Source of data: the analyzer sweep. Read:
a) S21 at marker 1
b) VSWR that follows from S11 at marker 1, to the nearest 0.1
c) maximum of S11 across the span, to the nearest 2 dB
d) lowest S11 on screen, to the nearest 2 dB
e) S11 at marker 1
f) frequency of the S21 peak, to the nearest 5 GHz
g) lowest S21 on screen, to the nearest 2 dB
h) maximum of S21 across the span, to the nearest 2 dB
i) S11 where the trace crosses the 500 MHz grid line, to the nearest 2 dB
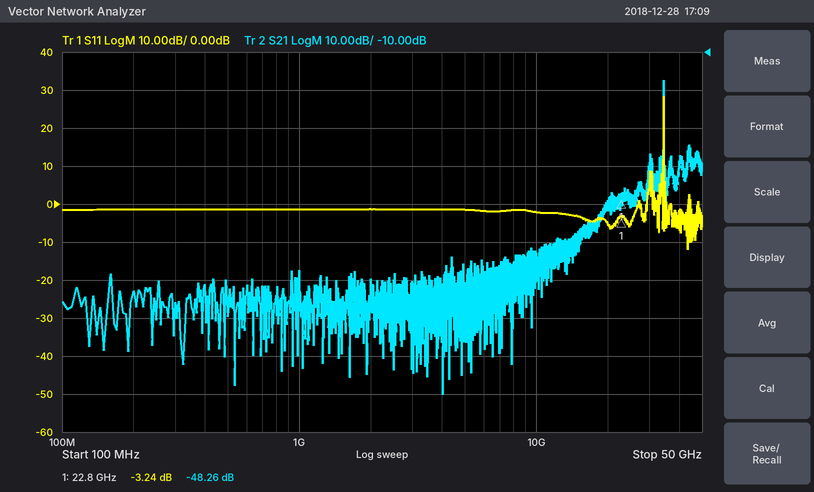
-48.26 dB
5.4
28 dB
-12 dB
-3.24 dB
35 GHz
-100 dB
-18 dB
-2 dB
